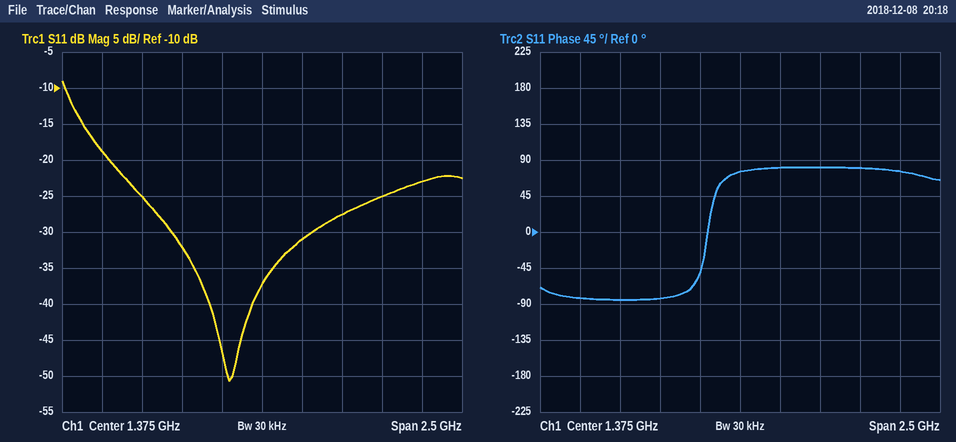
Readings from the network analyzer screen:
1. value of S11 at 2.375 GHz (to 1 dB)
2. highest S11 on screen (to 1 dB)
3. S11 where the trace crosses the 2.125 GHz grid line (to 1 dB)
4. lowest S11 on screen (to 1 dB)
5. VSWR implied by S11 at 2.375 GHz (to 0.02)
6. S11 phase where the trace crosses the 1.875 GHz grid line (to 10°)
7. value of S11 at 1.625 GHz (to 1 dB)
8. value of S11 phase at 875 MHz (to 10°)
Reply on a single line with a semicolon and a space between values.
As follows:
-23 dB; -9 dB; -25 dB; -51 dB; 1.16; 80°; -31 dB; -80°
